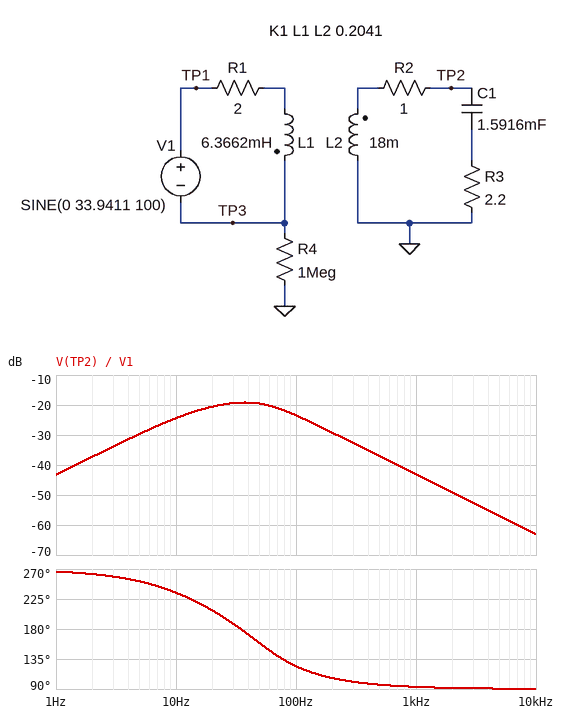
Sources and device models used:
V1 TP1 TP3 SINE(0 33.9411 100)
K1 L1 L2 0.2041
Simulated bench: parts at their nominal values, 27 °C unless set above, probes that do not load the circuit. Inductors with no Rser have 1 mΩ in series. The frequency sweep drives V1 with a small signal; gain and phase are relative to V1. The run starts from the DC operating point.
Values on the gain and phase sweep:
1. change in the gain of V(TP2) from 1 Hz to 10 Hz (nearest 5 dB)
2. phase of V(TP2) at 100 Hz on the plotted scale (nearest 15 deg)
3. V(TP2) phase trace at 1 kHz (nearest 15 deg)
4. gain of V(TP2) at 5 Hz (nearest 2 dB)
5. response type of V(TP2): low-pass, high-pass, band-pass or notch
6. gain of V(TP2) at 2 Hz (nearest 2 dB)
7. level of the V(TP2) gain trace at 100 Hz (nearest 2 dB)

20 dB
120 deg
90 deg
-30 dB
band-pass
-38 dB
-24 dB
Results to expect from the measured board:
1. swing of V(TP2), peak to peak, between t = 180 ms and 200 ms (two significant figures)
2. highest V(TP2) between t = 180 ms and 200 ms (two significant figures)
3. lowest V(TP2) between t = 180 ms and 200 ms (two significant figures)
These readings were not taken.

4.6 V
2.3 V
-2.3 V
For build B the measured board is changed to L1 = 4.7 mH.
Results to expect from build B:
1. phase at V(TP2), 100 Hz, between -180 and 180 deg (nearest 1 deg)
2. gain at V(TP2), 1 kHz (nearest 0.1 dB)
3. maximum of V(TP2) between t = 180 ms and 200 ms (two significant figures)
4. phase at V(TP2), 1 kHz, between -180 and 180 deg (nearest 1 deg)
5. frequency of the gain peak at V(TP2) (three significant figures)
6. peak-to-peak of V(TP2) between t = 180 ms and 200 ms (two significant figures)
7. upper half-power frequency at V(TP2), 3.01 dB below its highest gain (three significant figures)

148 deg
-37.3 dB
3.7 V
96 deg
57.1 Hz
7.4 V
127 Hz
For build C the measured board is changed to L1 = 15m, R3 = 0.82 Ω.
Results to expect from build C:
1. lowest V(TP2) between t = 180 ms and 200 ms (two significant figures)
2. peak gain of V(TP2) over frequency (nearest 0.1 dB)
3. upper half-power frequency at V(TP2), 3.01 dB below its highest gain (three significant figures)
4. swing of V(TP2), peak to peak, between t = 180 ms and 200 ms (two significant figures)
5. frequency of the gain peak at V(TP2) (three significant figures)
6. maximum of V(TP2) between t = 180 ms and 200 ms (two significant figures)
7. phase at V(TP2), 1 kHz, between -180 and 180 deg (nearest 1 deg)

-1.7 V
-16.5 dB
64.9 Hz
3.4 V
42.8 Hz
1.7 V
87 deg
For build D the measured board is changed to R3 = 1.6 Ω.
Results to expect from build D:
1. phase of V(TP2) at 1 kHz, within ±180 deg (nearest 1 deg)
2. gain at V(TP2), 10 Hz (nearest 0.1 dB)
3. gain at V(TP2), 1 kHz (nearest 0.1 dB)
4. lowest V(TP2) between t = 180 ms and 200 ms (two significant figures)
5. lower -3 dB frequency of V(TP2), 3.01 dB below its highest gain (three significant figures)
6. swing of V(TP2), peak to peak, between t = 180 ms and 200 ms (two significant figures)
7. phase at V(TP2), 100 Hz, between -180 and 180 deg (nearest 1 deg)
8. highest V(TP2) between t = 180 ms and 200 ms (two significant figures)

91 deg
-24.3 dB
-45.9 dB
-2.0 V
15.6 Hz
4.0 V
111 deg
2.0 V
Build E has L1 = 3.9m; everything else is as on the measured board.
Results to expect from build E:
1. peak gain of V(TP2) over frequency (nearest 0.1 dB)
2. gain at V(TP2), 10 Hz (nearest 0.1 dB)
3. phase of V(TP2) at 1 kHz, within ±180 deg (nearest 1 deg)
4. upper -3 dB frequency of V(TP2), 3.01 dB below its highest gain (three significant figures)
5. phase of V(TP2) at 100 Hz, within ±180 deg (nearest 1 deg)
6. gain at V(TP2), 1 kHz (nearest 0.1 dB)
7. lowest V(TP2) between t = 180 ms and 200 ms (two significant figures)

-17.8 dB
-29.9 dB
97 deg
140 Hz
153 deg
-36.5 dB
-3.8 V
